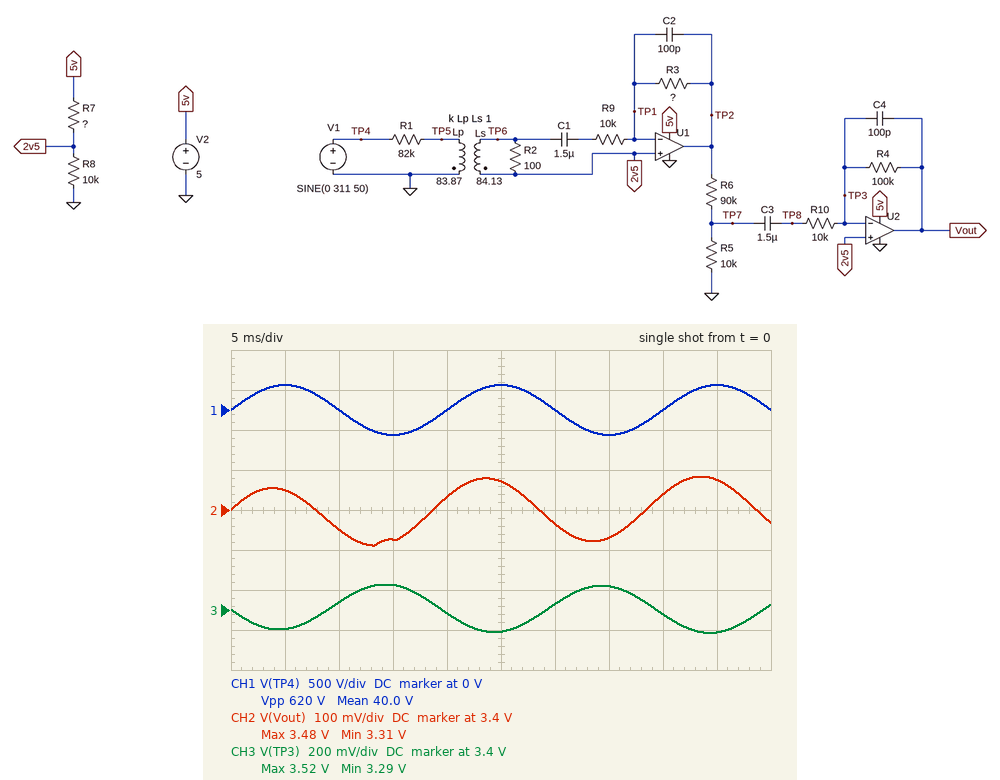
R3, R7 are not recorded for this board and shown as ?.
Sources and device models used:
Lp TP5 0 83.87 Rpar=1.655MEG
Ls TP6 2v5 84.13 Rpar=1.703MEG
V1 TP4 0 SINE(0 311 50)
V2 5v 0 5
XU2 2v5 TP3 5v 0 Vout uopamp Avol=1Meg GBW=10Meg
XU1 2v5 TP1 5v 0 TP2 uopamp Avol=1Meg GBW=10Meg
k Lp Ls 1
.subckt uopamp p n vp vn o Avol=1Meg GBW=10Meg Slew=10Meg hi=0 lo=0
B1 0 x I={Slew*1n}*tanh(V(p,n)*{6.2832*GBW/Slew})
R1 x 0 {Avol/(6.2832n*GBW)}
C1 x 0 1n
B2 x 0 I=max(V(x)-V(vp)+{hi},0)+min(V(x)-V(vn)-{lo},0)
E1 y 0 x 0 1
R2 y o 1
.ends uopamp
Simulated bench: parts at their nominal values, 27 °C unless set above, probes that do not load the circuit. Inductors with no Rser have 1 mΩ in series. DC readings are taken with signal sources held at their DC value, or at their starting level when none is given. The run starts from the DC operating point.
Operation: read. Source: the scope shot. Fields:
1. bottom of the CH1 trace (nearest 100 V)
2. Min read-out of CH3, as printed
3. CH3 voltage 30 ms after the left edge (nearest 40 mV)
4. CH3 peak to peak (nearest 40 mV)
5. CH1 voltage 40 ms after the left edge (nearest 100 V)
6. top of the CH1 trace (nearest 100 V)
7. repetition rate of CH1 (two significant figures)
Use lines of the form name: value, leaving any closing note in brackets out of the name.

bottom of the CH1 trace: -300 V
Min read-out of CH3, as printed: 3.29 V
CH3 voltage 30 ms after the left edge: 3.44 V
CH3 peak to peak: 240 mV
CH1 voltage 40 ms after the left edge: 0 V
top of the CH1 trace: 300 V
repetition rate of CH1: 50 Hz
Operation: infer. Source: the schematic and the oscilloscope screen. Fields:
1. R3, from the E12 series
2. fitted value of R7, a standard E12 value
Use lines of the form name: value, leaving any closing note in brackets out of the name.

R3, from the E12 series: 39 kΩ
fitted value of R7, a standard E12 value: 4.7 kΩ
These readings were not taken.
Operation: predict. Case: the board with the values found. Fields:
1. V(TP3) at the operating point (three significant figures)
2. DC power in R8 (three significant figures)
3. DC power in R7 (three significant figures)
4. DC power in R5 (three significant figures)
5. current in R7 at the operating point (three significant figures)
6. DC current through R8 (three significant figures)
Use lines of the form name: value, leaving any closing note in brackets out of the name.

V(TP3) at the operating point: 3.40 V
DC power in R8: 1.16 mW
DC power in R7: 544 µW
DC power in R5: 11.6 µW
current in R7 at the operating point: 340 µA
DC current through R8: 340 µA
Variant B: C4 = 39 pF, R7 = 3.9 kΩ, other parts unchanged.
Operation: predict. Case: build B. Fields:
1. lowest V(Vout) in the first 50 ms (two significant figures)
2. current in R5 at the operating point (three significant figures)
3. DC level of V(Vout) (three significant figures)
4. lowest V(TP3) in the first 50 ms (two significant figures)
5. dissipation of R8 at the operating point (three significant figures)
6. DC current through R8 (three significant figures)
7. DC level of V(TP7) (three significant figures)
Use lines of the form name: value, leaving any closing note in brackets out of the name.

lowest V(Vout) in the first 50 ms: 3.4 V
current in R5 at the operating point: 36.0 µA
DC level of V(Vout): 3.60 V
lowest V(TP3) in the first 50 ms: 3.5 V
dissipation of R8 at the operating point: 1.29 mW
DC current through R8: 360 µA
DC level of V(TP7): 360 mV
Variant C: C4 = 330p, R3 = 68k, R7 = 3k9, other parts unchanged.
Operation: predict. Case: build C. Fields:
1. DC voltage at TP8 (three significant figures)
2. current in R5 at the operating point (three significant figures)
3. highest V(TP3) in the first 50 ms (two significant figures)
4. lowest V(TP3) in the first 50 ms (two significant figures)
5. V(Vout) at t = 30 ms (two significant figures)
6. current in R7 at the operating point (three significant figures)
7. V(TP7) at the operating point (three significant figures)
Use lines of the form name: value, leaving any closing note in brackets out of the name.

DC voltage at TP8: 3.60 V
current in R5 at the operating point: 36.0 µA
highest V(TP3) in the first 50 ms: 3.7 V
lowest V(TP3) in the first 50 ms: 3.5 V
V(Vout) at t = 30 ms: 3.3 V
current in R7 at the operating point: 360 µA
V(TP7) at the operating point: 360 mV
